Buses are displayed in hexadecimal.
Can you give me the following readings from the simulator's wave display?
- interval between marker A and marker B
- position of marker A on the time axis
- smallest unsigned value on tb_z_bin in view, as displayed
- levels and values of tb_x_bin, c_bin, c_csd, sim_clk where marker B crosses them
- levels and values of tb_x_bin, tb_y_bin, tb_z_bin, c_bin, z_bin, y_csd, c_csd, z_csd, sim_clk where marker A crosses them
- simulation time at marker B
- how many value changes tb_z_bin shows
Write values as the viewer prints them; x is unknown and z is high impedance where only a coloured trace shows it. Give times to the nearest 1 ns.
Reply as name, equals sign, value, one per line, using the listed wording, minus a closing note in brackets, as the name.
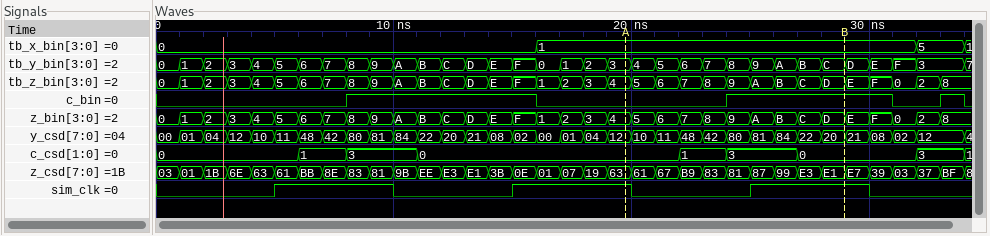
interval between marker A and marker B = 9 ns
position of marker A on the time axis = 20 ns
smallest unsigned value on tb_z_bin in view, as displayed = 0
levels and values of tb_x_bin, c_bin, c_csd, sim_clk where marker B crosses them = tb_x_bin=1, c_bin=1, c_csd=0, sim_clk=1
levels and values of tb_x_bin, tb_y_bin, tb_z_bin, c_bin, z_bin, y_csd, c_csd, z_csd, sim_clk where marker A crosses them = tb_x_bin=1, tb_y_bin=3, tb_z_bin=4, c_bin=0, z_bin=4, y_csd=12, c_csd=0, z_csd=63, sim_clk=1
simulation time at marker B = 29 ns
how many value changes tb_z_bin shows = 33
